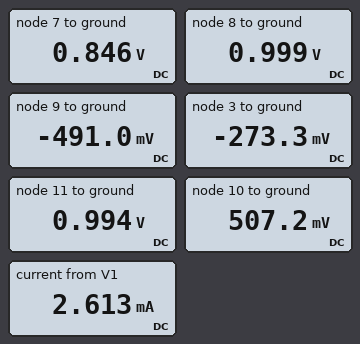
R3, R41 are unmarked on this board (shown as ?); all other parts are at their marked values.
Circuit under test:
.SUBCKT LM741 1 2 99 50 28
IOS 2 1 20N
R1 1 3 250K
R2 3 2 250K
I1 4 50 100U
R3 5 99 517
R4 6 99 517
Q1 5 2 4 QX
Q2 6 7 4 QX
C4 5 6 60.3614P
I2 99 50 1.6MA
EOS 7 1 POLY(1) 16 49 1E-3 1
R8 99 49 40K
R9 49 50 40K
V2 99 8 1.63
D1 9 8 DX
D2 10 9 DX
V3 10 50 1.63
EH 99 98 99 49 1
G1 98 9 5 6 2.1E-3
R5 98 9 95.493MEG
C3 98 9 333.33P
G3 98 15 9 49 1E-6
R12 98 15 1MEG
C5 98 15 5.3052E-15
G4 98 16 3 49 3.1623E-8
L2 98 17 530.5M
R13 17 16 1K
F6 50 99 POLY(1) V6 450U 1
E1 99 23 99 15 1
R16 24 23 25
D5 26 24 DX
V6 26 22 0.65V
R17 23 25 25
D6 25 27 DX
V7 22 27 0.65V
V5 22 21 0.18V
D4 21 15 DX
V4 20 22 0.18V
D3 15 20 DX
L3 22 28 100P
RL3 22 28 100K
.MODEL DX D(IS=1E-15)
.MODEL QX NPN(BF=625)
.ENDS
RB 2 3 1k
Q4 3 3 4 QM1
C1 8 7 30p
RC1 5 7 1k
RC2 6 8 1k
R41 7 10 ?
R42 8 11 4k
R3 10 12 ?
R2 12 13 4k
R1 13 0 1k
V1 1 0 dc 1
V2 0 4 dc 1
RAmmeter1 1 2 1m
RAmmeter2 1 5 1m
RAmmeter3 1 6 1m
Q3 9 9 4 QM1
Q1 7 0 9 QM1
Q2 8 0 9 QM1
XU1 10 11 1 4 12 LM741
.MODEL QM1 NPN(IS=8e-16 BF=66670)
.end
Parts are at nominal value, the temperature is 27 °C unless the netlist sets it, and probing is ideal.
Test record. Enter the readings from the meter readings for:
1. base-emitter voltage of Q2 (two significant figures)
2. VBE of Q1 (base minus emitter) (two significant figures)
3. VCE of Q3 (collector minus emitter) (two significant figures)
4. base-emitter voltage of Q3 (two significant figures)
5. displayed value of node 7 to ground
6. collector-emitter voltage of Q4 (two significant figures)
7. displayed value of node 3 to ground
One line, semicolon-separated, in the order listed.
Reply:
490 mV; 490 mV; 510 mV; 510 mV; 0.846 V; 730 mV; -273.3 mV
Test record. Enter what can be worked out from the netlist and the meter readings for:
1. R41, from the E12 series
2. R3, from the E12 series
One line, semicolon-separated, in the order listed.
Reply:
2.2 kΩ; 3.3 kΩ
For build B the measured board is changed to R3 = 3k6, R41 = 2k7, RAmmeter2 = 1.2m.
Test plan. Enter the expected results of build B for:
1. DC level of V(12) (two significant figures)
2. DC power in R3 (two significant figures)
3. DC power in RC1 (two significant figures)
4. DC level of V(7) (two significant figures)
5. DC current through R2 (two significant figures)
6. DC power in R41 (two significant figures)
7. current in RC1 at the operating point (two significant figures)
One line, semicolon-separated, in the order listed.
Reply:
-6.5 mV; 69 µW; 19 µW; 860 mV; 1.3 µA; 51 µW; 140 µA
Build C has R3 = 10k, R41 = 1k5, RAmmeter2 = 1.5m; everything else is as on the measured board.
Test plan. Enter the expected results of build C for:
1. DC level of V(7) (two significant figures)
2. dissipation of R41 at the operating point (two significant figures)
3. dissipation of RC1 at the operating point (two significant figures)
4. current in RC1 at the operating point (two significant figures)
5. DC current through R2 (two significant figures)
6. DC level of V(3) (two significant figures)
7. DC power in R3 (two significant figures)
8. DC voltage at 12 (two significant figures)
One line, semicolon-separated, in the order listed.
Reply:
920 mV; 9.8 µW; 6.6 µW; 81 µA; 3.0 µA; -270 mV; 66 µW; -15 mV
